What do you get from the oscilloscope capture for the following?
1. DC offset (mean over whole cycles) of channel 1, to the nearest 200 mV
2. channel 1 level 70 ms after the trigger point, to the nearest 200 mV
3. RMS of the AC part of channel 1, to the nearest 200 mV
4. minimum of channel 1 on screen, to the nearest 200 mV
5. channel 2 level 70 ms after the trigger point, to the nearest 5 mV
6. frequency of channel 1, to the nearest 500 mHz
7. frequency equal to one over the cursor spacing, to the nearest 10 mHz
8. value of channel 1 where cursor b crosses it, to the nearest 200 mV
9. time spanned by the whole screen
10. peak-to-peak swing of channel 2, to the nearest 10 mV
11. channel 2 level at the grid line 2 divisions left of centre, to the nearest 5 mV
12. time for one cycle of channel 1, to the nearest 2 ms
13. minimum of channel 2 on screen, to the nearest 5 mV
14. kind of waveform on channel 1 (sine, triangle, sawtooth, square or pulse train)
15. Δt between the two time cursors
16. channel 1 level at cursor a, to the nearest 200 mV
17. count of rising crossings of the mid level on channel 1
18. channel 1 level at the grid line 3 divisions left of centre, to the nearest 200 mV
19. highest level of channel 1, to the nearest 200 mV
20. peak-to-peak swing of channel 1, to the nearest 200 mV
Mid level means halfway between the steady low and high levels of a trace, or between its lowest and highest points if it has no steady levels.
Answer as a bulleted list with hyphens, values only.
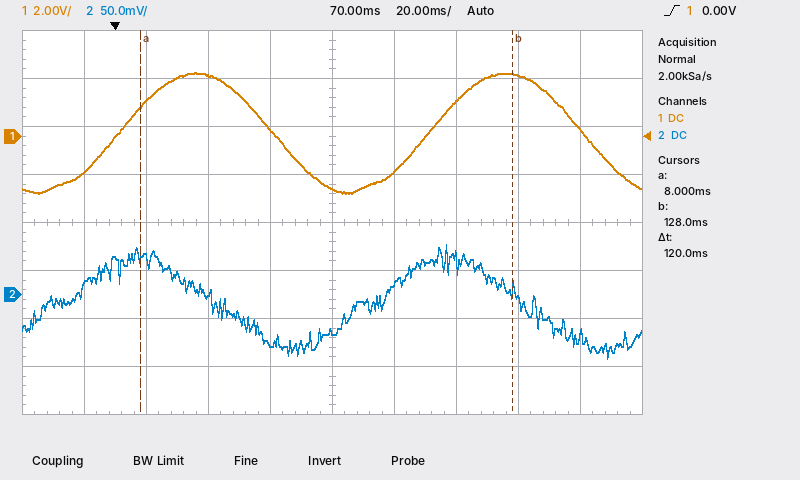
- 200 mV
- -2.2 V
- 1.8 V
- -2.4 V
- -40 mV
- 10.0 Hz
- 8.33 Hz
- 2.6 V
- 200 ms
- 120 mV
- 0 mV
- 100 ms
- -65 mV
- sine
- 120 ms
- 1.2 V
- 2
- 1.4 V
- 2.6 V
- 5.0 V
